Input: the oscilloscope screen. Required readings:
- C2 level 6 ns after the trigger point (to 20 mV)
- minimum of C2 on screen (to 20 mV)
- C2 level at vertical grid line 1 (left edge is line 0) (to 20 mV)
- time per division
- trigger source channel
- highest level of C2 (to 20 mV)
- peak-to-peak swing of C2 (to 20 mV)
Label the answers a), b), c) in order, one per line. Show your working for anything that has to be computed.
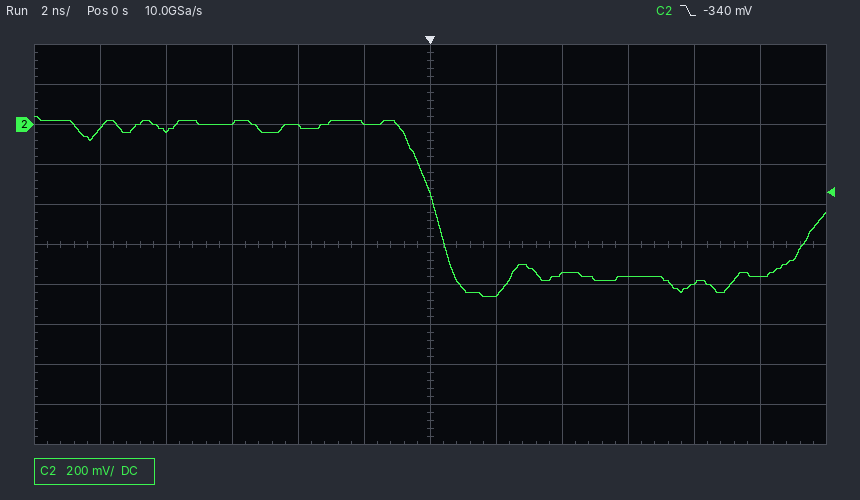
a) -760 mV
b) -860 mV
c) -20 mV
d) 2 ns
e) C2
f) 40 mV
g) 40 mV − (-860 mV) = 900 mV
